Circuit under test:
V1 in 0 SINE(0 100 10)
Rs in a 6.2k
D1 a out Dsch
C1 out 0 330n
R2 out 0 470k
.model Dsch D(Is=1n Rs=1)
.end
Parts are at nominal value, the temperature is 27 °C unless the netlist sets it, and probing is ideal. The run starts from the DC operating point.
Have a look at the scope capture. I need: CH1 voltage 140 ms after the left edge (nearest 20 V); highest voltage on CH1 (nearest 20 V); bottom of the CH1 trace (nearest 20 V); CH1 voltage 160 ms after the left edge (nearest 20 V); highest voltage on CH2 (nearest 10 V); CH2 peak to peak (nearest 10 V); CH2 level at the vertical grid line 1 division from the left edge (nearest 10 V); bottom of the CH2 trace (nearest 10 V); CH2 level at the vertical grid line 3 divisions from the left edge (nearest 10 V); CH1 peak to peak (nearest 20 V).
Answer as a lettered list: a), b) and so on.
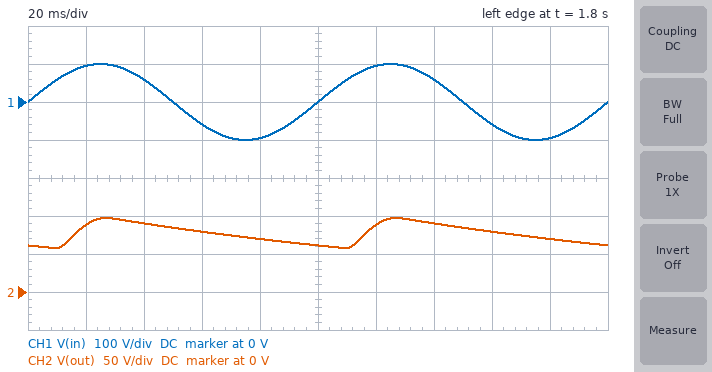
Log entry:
a) 60 V
b) 100 V
c) -100 V
d) -60 V
e) 100 V
f) 40 V
g) 90 V
h) 60 V
i) 80 V
j) 200 V
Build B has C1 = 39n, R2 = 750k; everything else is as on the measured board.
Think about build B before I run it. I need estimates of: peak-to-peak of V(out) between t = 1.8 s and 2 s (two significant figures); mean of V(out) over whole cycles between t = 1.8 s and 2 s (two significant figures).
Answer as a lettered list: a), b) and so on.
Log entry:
a) 90 V
b) 46 V
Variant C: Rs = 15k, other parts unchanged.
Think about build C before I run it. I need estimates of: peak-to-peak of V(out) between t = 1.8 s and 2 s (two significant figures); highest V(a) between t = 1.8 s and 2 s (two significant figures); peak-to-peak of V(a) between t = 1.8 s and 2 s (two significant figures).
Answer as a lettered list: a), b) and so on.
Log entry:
a) 37 V
b) 93 V
c) 190 V
